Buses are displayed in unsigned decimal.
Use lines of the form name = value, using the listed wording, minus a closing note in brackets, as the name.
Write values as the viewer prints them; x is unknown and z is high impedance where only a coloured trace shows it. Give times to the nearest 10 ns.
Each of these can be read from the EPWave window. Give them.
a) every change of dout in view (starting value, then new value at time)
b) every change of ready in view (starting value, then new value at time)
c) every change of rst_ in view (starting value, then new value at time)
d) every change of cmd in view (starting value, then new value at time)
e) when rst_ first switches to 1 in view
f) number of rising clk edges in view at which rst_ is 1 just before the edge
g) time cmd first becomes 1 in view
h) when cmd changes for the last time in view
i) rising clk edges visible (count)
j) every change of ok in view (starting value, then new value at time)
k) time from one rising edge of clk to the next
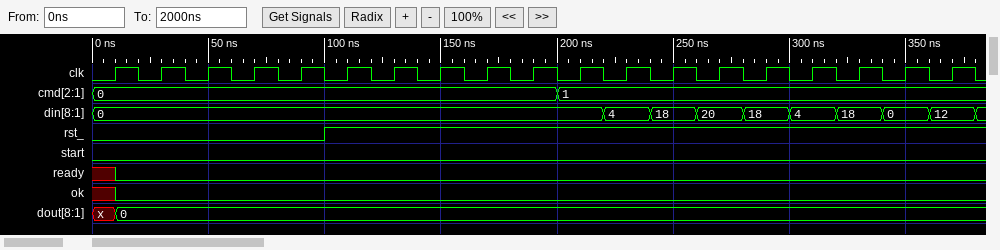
every change of dout in view = x, 0 at 10 ns
every change of ready in view = x, 0 at 10 ns
every change of rst_ in view = 0, 1 at 100 ns
every change of cmd in view = 0, 1 at 200 ns
when rst_ first switches to 1 in view = 100 ns
number of rising clk edges in view at which rst_ is 1 just before the edge = 14
time cmd first becomes 1 in view = 200 ns
when cmd changes for the last time in view = 200 ns
rising clk edges visible = 19
every change of ok in view = x, 0 at 10 ns
time from one rising edge of clk to the next = 20 ns
